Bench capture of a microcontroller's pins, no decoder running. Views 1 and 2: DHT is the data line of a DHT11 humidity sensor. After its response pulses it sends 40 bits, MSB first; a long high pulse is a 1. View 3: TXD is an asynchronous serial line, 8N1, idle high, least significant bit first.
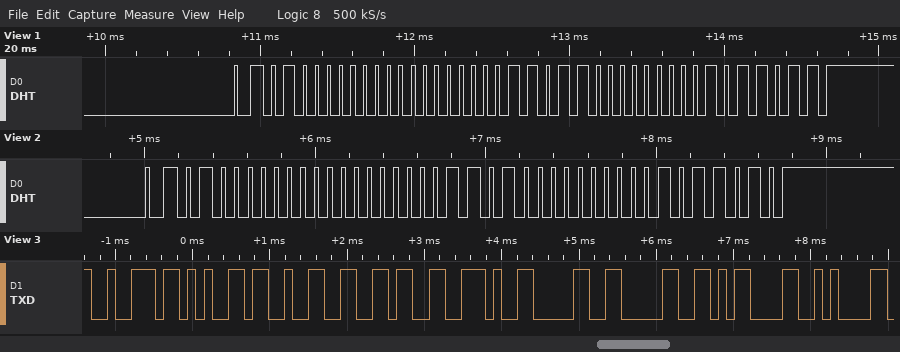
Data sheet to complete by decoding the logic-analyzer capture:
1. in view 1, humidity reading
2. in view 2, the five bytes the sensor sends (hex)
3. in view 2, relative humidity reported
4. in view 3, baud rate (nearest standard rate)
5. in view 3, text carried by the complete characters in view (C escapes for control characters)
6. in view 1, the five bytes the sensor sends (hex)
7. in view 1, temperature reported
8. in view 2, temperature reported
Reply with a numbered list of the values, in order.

1. 64 %
2. 40 00 1A 00 5A
3. 64 %
4. 9600 baud
5. "re26.00\r\n"
6. 40 00 1B 00 5B
7. 27.0 °C
8. 26.0 °C
